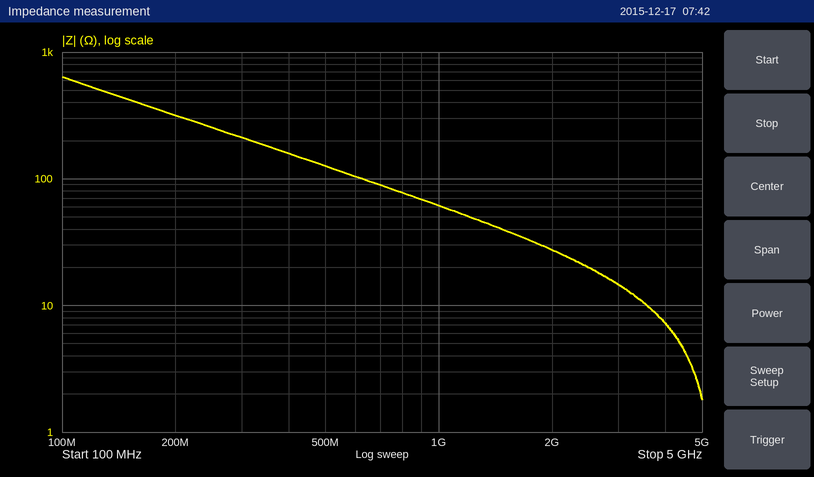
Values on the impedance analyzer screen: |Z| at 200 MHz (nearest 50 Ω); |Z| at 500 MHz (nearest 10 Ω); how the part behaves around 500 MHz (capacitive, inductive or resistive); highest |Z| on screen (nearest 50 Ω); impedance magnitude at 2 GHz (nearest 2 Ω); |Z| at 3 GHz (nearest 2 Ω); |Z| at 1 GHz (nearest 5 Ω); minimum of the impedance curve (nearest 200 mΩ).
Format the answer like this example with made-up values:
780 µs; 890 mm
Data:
300 Ω; 130 Ω; capacitive; 650 Ω; 28 Ω; 14 Ω; 60 Ω; 1.8 Ω
